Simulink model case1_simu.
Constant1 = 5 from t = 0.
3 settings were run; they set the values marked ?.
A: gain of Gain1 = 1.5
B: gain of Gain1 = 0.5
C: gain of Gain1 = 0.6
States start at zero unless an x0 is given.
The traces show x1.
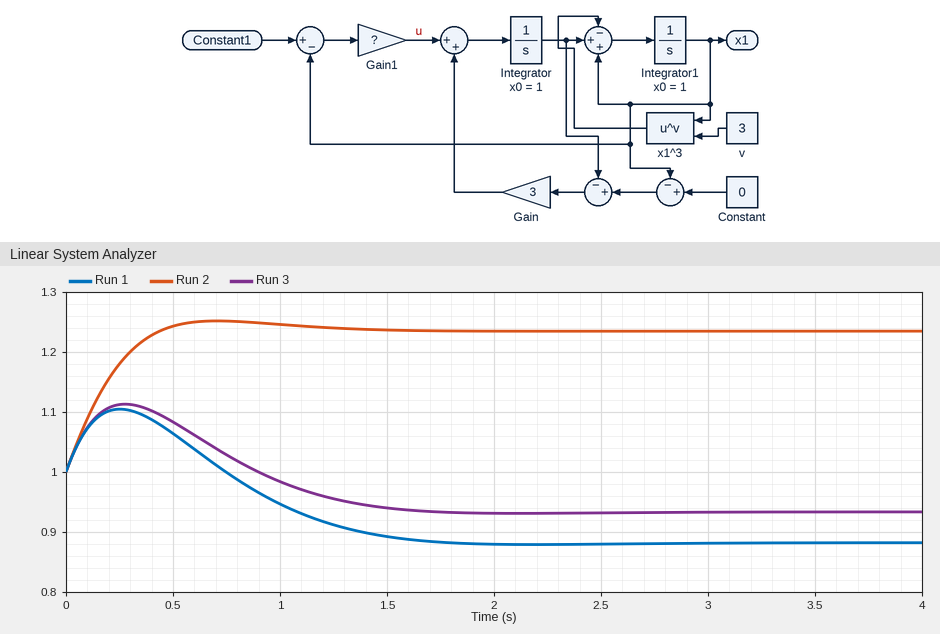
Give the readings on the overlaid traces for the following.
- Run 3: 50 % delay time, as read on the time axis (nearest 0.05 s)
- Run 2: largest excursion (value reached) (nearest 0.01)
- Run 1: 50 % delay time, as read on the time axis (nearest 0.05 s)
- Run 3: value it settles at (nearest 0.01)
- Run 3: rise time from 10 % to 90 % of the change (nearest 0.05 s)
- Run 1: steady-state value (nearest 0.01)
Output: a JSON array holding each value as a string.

["1.15 s", "1.25", "1.05 s", "0.93", "0.55 s", "0.88"]
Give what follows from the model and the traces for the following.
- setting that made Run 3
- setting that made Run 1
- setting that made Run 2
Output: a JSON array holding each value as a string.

["C", "B", "A"]
